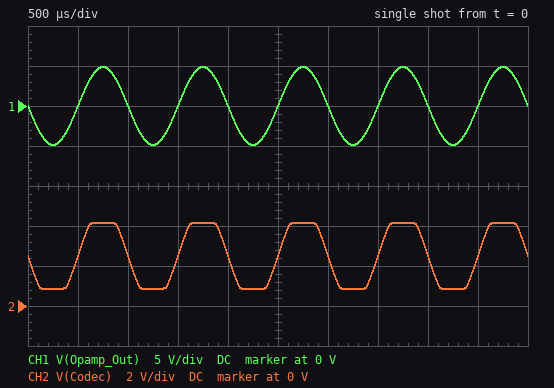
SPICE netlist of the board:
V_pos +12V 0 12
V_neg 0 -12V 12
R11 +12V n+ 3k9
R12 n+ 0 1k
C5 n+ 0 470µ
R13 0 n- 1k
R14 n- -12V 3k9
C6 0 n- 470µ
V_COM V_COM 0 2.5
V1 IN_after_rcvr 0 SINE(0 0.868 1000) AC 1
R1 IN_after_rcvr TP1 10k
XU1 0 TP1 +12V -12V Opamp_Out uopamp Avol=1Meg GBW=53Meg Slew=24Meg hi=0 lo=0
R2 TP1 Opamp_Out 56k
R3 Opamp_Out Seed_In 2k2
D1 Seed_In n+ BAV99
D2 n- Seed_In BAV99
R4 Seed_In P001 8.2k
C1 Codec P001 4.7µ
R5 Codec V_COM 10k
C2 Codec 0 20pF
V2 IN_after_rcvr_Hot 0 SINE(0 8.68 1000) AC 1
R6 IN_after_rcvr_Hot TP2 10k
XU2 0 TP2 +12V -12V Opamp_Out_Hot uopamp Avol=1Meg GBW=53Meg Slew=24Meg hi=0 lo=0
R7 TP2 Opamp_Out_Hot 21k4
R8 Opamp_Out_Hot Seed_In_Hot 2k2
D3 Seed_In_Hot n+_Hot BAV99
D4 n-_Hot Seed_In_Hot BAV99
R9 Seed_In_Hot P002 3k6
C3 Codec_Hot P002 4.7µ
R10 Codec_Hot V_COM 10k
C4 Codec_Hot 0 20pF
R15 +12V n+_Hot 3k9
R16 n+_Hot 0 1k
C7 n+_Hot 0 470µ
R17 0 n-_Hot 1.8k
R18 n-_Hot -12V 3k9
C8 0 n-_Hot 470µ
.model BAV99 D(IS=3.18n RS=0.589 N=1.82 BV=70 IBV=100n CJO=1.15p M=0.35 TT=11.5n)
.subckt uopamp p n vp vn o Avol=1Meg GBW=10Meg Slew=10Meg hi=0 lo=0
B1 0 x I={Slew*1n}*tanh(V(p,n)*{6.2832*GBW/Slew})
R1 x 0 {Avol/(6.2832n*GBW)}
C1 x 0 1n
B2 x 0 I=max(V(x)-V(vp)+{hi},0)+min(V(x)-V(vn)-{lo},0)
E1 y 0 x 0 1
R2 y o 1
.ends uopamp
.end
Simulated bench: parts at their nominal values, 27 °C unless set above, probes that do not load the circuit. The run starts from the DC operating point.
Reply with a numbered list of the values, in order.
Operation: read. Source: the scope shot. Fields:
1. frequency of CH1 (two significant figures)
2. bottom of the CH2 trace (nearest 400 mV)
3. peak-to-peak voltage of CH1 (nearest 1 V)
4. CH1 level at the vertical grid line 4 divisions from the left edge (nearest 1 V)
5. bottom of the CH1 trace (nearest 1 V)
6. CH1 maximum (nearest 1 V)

1. 1.0 kHz
2. 800 mV
3. 10 V
4. 0 V
5. -5 V
6. 5 V
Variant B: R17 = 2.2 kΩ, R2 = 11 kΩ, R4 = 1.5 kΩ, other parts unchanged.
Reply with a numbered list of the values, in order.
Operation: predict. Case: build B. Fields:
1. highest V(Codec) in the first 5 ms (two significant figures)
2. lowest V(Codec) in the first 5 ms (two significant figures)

1. 3.2 V
2. 1.8 V
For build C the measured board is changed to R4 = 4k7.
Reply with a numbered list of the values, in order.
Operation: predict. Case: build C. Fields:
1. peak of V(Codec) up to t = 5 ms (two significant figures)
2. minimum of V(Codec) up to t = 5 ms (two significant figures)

1. 4.6 V
2. 450 mV
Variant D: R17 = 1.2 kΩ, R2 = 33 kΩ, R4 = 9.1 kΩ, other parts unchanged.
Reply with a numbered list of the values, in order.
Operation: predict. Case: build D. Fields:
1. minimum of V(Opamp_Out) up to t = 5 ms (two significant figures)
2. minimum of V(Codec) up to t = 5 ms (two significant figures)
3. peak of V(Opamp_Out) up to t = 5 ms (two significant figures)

1. -2.9 V
2. 1.2 V
3. 2.9 V
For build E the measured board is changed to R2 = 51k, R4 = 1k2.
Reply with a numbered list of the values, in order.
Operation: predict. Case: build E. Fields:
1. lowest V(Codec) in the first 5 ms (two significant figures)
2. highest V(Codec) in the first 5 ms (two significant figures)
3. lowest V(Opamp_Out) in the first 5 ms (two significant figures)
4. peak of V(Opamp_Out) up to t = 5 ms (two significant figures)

1. -170 mV
2. 5.2 V
3. -4.4 V
4. 4.4 V
